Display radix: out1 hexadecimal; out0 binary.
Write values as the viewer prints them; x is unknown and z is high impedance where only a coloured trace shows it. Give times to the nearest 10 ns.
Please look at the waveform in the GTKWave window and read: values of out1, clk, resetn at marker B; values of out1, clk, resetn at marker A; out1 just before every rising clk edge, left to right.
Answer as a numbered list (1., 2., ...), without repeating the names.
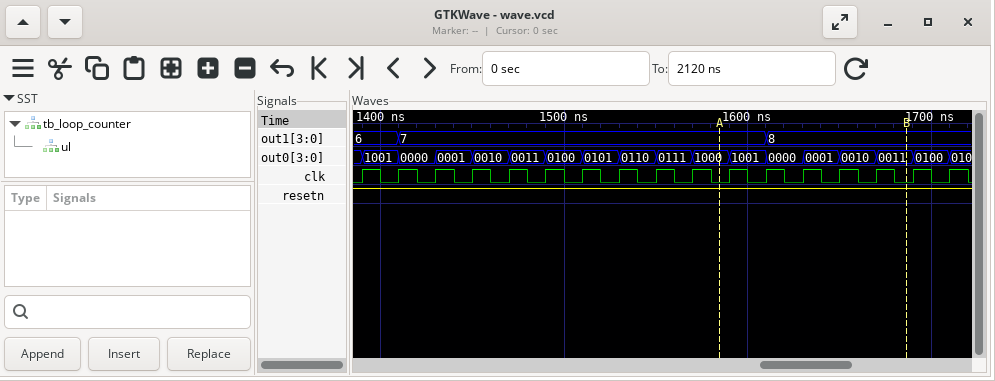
1. out1=8, clk=0, resetn=1
2. out1=7, clk=0, resetn=1
3. 6, 6, 7, 7, 7, 7, 7, 7, 7, 7, 7, 7, 8, 8, 8, 8, 8
